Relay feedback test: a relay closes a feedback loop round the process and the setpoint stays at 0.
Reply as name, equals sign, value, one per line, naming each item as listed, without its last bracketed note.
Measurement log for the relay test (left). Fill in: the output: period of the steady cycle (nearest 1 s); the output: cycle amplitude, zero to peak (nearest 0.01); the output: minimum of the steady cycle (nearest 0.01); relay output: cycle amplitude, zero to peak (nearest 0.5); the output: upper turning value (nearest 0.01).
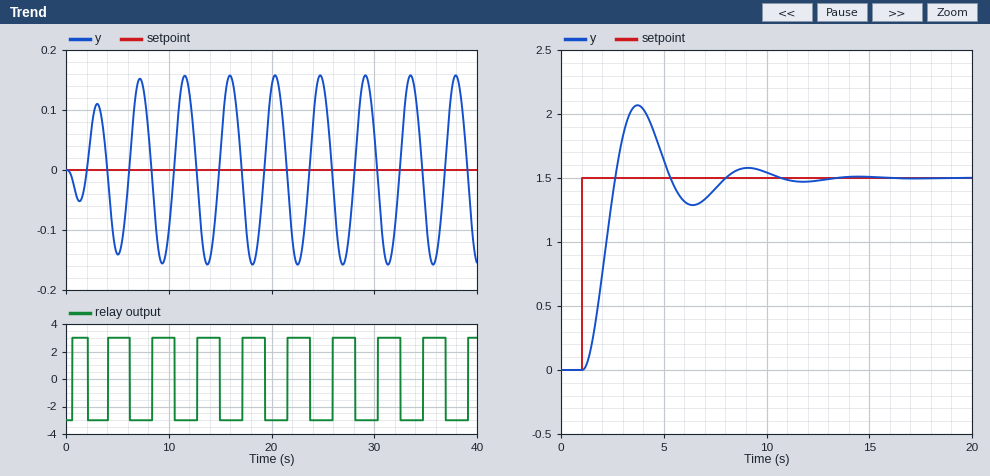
the output: period of the steady cycle = 4 s
the output: cycle amplitude, zero to peak = 0.16
the output: minimum of the steady cycle = -0.16
relay output: cycle amplitude, zero to peak = 3.0
the output: upper turning value = 0.16
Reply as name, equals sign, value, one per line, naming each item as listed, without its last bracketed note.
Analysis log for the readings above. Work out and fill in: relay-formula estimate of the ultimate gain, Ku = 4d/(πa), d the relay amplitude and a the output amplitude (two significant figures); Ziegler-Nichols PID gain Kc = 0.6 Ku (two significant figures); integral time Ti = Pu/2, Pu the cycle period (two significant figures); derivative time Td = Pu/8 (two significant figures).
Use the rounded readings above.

relay-formula estimate of the ultimate gain, Ku = 4d/(πa), d the relay amplitude and a the output amplitude = 24
Ziegler-Nichols PID gain Kc = 0.6 Ku = 14
integral time Ti = Pu/2, Pu the cycle period = 2.0 s
derivative time Td = Pu/8 = 0.50 s
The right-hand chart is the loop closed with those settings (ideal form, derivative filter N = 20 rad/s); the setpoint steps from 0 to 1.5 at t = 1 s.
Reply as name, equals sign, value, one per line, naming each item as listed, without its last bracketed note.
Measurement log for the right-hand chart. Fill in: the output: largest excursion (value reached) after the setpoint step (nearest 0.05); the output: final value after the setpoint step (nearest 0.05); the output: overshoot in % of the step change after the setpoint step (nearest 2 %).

the output: largest excursion (value reached) after the setpoint step = 2.05
the output: final value after the setpoint step = 1.50
the output: overshoot in % of the step change after the setpoint step = 38 %
